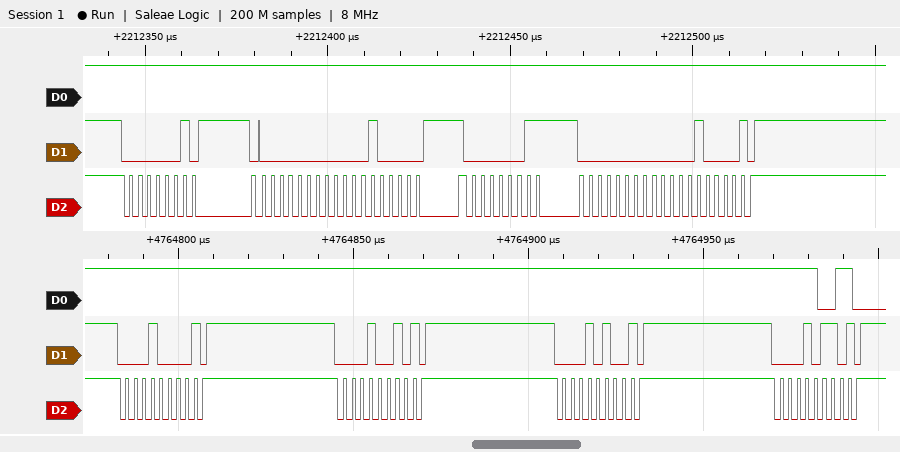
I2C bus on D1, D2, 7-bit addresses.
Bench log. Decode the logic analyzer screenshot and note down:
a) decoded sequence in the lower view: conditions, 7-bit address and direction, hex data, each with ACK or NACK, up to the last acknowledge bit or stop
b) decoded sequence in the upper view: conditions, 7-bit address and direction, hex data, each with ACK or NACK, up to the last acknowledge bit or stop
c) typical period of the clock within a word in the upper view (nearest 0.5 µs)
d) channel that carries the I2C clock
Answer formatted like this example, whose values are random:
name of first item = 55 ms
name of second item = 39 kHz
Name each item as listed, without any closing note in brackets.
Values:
decoded sequence in the lower view: conditions, 7-bit address and direction, hex data, each with ACK or NACK, up to the last acknowledge bit or stop = start, address 08 write NACK, stop, start, address 09 write NACK, stop, start, address 0A write NACK, stop, start, address 0B write NACK, stop
decoded sequence in the upper view: conditions, 7-bit address and direction, hex data, each with ACK or NACK, up to the last acknowledge bit or stop = start, address 01 write ACK, 00 ACK, 10 ACK, repeated start, address 01 read ACK, 00 ACK, 10 NACK, stop
typical period of the clock within a word in the upper view = 2.5 µs
channel that carries the I2C clock = D2
